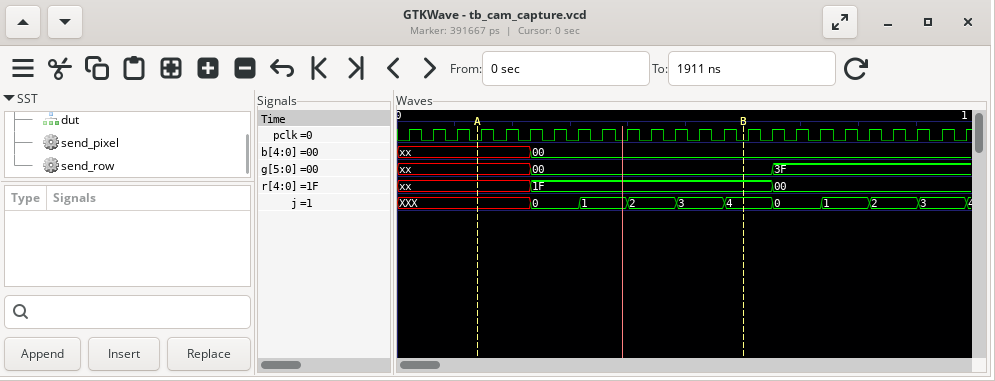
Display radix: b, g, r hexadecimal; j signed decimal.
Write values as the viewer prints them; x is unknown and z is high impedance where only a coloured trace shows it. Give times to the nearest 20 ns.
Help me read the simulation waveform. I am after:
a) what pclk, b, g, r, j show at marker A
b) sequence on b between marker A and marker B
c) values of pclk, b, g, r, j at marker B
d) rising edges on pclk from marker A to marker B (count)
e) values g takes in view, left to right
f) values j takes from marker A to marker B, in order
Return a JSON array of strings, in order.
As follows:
["pclk=0, b=xx, g=xx, r=xx, j=XXX", "xx, 00", "pclk=0, b=00, g=00, r=1F, j=4", "11", "xx, 00, 3F", "XXX, 0, 1, 2, 3, 4"]
